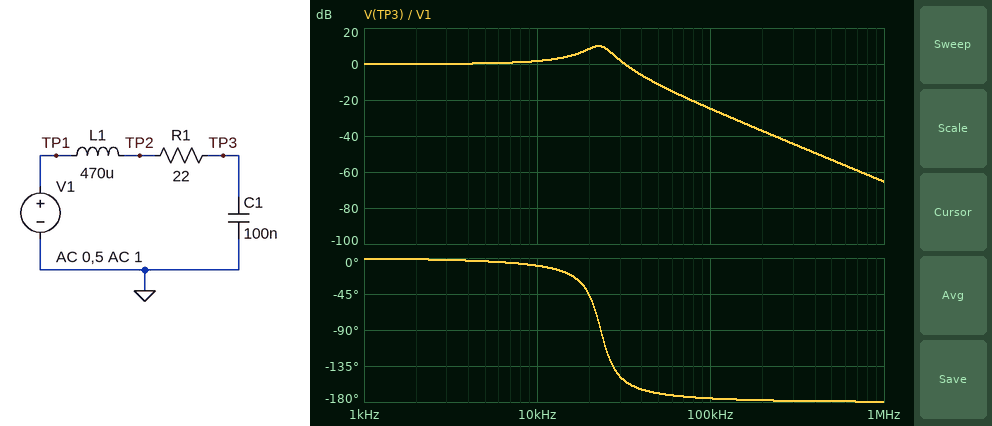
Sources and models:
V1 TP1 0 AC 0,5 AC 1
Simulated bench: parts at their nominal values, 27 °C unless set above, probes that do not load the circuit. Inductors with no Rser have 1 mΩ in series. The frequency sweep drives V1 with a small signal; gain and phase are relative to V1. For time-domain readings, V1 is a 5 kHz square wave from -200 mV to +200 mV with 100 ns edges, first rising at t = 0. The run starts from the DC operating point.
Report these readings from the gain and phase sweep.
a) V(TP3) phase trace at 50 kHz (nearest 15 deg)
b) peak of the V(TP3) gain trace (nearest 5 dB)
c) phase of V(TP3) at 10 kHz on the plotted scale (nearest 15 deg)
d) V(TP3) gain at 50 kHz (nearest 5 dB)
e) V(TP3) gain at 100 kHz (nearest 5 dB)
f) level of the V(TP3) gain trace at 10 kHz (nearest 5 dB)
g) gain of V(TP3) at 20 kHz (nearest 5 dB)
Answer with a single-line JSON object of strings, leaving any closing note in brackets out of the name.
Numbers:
{"V(TP3) phase trace at 50 kHz": "-165 deg", "peak of the V(TP3) gain trace": "10 dB", "phase of V(TP3) at 10 kHz on the plotted scale": "-15 deg", "V(TP3) gain at 50 kHz": "-10 dB", "V(TP3) gain at 100 kHz": "-25 dB", "level of the V(TP3) gain trace at 10 kHz": "0 dB", "gain of V(TP3) at 20 kHz": "10 dB"}
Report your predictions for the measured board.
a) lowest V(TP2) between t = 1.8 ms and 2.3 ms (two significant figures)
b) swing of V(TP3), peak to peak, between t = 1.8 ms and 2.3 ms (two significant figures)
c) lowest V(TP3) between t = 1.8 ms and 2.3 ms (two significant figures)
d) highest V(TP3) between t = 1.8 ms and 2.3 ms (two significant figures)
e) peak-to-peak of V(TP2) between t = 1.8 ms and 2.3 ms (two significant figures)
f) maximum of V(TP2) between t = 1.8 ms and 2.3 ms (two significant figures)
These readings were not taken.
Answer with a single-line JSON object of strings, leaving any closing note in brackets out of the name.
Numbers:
{"lowest V(TP2) between t = 1.8 ms and 2.3 ms": "-450 mV", "swing of V(TP3), peak to peak, between t = 1.8 ms and 2.3 ms": "880 mV", "lowest V(TP3) between t = 1.8 ms and 2.3 ms": "-440 mV", "highest V(TP3) between t = 1.8 ms and 2.3 ms": "440 mV", "peak-to-peak of V(TP2) between t = 1.8 ms and 2.3 ms": "910 mV", "maximum of V(TP2) between t = 1.8 ms and 2.3 ms": "450 mV"}
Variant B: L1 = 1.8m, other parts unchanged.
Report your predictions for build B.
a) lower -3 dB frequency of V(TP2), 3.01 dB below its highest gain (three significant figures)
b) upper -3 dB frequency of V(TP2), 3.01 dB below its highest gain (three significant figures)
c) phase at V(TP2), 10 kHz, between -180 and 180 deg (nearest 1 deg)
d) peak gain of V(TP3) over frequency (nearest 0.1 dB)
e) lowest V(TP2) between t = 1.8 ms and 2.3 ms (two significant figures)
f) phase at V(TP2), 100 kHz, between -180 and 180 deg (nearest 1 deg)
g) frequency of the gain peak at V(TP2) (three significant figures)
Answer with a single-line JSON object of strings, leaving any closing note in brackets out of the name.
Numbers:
{"lower -3 dB frequency of V(TP2), 3.01 dB below its highest gain": "10.8 kHz", "upper -3 dB frequency of V(TP2), 3.01 dB below its highest gain": "12.7 kHz", "phase at V(TP2), 10 kHz, between -180 and 180 deg": "-18 deg", "peak gain of V(TP3) over frequency": "15.7 dB", "lowest V(TP2) between t = 1.8 ms and 2.3 ms": "-430 mV", "phase at V(TP2), 100 kHz, between -180 and 180 deg": "-125 deg", "frequency of the gain peak at V(TP2)": "11.8 kHz"}
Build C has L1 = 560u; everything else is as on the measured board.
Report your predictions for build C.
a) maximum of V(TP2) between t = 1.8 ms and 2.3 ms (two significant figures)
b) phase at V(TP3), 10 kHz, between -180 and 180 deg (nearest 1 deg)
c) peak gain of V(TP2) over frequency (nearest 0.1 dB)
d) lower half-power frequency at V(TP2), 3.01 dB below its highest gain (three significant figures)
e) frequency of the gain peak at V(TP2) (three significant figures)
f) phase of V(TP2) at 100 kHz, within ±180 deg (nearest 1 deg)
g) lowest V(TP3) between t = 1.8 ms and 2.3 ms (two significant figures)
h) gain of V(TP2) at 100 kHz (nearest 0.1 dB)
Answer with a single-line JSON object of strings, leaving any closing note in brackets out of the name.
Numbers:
{"maximum of V(TP2) between t = 1.8 ms and 2.3 ms": "430 mV", "phase at V(TP3), 10 kHz, between -180 and 180 deg": "-10 deg", "peak gain of V(TP2) over frequency": "11.1 dB", "lower half-power frequency at V(TP2), 3.01 dB below its highest gain": "17.4 kHz", "frequency of the gain peak at V(TP2)": "20.8 kHz", "phase of V(TP2) at 100 kHz, within ±180 deg": "-122 deg", "lowest V(TP3) between t = 1.8 ms and 2.3 ms": "-420 mV", "gain of V(TP2) at 100 kHz": "-21.9 dB"}
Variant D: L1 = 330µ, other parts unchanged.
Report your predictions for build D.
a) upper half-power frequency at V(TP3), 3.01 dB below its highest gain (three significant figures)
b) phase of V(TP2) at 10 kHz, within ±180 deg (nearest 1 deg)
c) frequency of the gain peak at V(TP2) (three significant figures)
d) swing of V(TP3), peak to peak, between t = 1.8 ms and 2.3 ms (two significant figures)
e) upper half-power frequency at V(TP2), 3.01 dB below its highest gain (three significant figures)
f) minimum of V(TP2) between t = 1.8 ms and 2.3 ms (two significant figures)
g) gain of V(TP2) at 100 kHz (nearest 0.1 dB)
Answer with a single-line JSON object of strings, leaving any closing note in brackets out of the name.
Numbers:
{"upper half-power frequency at V(TP3), 3.01 dB below its highest gain": "31.6 kHz", "phase of V(TP2) at 10 kHz, within ±180 deg": "-1 deg", "frequency of the gain peak at V(TP2)": "26.8 kHz", "swing of V(TP3), peak to peak, between t = 1.8 ms and 2.3 ms": "840 mV", "upper half-power frequency at V(TP2), 3.01 dB below its highest gain": "31.8 kHz", "minimum of V(TP2) between t = 1.8 ms and 2.3 ms": "-440 mV", "gain of V(TP2) at 100 kHz": "-17.0 dB"}
